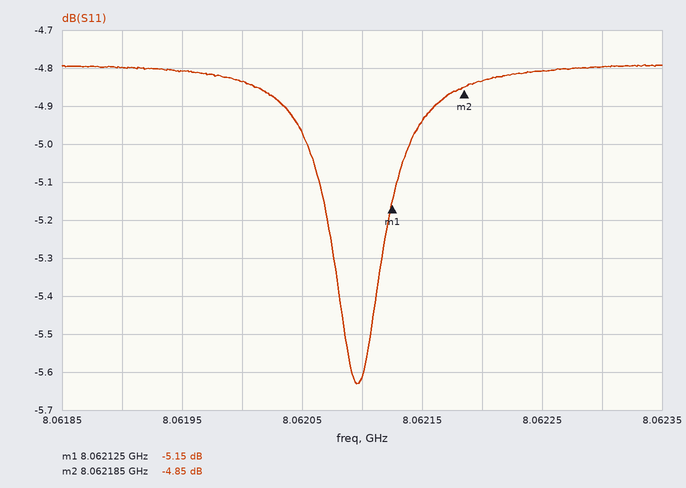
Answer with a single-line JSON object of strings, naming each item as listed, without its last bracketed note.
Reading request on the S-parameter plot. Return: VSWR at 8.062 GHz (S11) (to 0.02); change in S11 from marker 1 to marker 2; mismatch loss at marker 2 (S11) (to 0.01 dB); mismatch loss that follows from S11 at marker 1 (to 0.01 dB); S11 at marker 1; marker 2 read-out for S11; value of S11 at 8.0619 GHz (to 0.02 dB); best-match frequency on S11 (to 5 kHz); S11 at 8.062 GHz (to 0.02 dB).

{"VSWR at 8.062 GHz (S11)": "3.68", "change in S11 from marker 1 to marker 2": "0.30 dB", "mismatch loss at marker 2 (S11)": "1.72 dB", "mismatch loss that follows from S11 at marker 1": "1.58 dB", "S11 at marker 1": "-5.15 dB", "marker 2 read-out for S11": "-4.85 dB", "value of S11 at 8.0619 GHz": "-4.80 dB", "best-match frequency on S11": "8.062095 GHz", "S11 at 8.062 GHz": "-4.84 dB"}
